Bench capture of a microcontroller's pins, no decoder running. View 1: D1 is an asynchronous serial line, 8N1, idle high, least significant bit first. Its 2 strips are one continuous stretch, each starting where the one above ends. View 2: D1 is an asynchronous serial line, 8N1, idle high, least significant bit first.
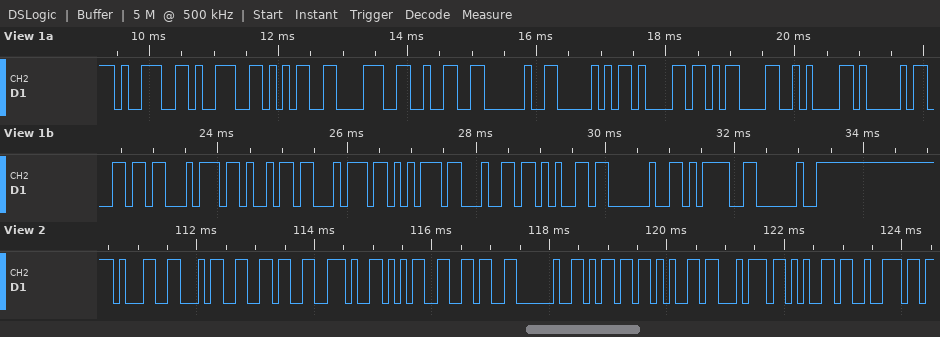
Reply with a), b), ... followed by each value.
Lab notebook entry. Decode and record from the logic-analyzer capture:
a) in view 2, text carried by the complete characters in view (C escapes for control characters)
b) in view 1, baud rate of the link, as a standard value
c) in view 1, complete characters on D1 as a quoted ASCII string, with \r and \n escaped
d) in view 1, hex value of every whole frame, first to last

a) "146.56 meter"
b) 9600 baud
c) "99582 Pa\r\nAltitude = "
d) 39 39 35 38 32 20 50 61 0D 0A 41 6C 74 69 74 75 64 65 20 3D 20
